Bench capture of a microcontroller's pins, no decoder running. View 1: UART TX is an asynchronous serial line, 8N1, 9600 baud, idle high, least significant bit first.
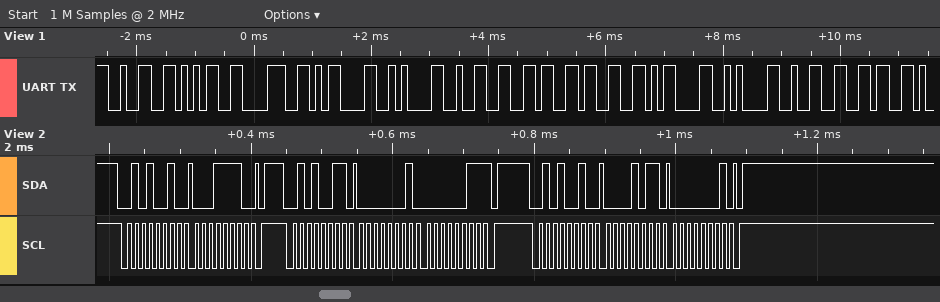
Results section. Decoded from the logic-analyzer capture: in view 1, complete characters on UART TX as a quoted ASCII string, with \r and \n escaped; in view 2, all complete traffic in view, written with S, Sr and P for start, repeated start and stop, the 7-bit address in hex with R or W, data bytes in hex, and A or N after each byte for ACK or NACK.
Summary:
"258\r\n263\r\n26"
S 29W A 1E A P S 29R A 01 A 03 N P S 29W A 0B A 01 A P
